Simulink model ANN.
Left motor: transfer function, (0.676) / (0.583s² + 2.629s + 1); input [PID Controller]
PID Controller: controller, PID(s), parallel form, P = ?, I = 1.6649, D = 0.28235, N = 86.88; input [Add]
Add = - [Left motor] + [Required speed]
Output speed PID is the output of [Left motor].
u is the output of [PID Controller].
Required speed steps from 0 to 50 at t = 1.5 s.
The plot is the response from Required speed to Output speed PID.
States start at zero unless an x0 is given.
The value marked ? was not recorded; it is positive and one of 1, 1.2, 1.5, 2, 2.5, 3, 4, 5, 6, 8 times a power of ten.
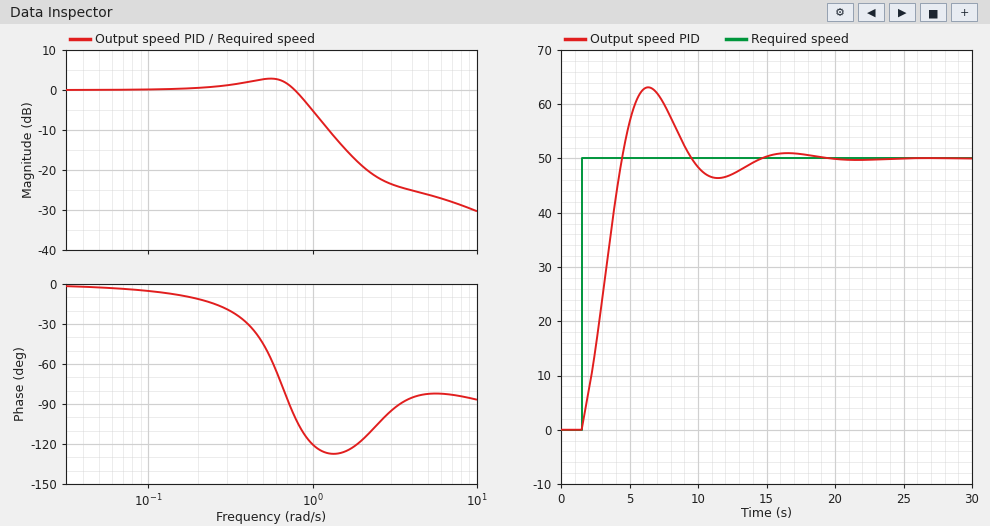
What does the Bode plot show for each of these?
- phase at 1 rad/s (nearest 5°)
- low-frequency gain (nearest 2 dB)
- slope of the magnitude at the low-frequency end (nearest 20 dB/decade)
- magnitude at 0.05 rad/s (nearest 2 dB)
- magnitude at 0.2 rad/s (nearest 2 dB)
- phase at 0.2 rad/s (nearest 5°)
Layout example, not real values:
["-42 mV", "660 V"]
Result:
["-120°", "0 dB", "0 dB/decade", "0 dB", "0 dB", "-10°"]
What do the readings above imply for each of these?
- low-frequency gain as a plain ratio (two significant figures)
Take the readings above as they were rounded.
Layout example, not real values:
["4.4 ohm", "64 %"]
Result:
["1.0"]
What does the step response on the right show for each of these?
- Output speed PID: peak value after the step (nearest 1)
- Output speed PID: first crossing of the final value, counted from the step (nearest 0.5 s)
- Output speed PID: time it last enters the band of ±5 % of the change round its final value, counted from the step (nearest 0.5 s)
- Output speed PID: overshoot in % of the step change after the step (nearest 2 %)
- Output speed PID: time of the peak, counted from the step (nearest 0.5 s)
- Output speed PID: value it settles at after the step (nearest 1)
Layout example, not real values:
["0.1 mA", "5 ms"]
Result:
["63", "3.0 s", "11.5 s", "26 %", "5.0 s", "50"]
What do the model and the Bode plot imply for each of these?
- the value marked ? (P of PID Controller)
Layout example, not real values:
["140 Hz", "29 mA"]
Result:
["0.8"]
